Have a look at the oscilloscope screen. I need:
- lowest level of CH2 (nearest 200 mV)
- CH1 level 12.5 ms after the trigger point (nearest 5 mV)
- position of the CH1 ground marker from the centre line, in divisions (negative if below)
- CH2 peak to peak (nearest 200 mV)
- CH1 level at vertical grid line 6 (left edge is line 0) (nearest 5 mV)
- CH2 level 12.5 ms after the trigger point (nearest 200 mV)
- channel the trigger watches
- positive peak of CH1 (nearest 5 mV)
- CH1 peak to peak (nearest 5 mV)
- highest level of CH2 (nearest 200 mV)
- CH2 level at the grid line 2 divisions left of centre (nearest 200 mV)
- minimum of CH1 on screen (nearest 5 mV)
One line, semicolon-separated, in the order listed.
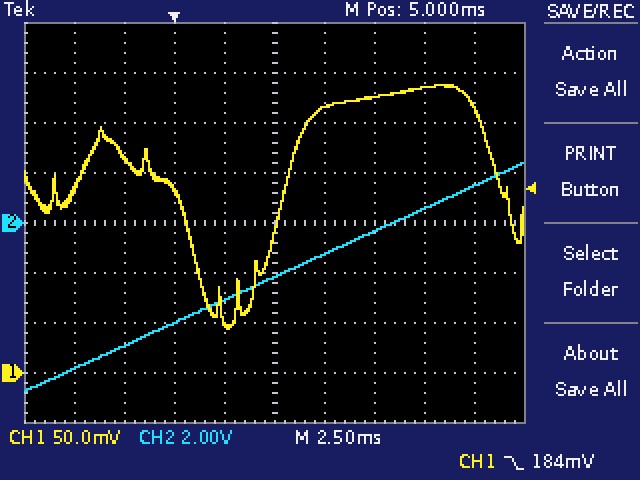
-6.8 V; 285 mV; -3.0 div; 9.2 V; 265 mV; 600 mV; CH1; 290 mV; 245 mV; 2.4 V; -4.0 V; 45 mV
